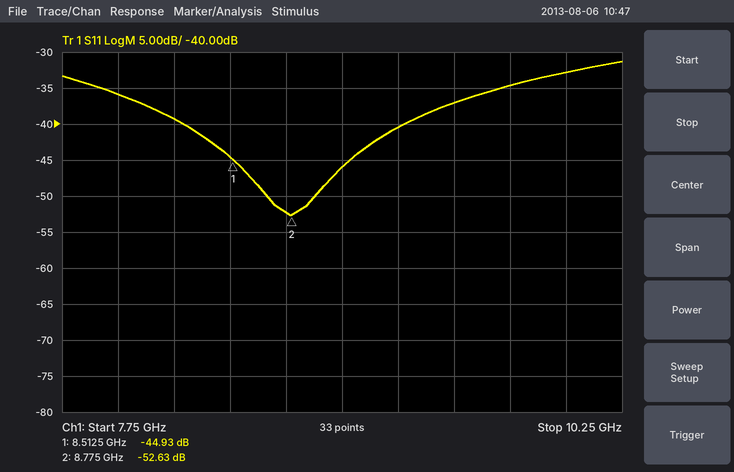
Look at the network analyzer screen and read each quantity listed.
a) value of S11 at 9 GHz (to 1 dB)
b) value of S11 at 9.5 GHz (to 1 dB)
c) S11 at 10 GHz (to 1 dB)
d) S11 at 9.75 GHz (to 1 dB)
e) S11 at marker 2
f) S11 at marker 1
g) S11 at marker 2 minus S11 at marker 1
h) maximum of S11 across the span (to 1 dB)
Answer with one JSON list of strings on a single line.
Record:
["-46 dB", "-37 dB", "-33 dB", "-35 dB", "-52.63 dB", "-44.93 dB", "-7.70 dB", "-31 dB"]
